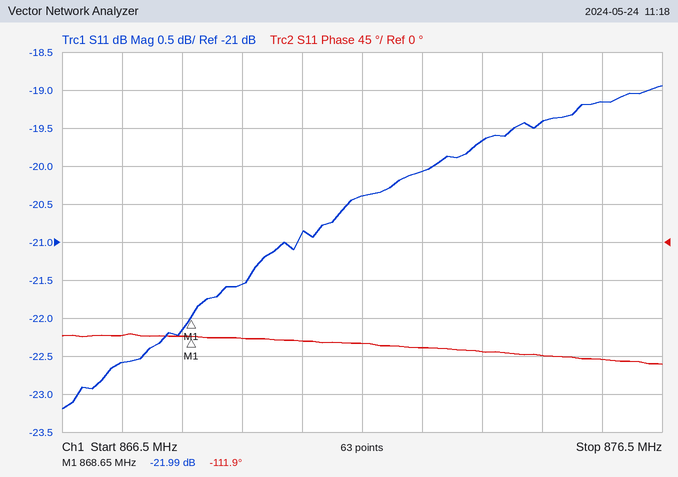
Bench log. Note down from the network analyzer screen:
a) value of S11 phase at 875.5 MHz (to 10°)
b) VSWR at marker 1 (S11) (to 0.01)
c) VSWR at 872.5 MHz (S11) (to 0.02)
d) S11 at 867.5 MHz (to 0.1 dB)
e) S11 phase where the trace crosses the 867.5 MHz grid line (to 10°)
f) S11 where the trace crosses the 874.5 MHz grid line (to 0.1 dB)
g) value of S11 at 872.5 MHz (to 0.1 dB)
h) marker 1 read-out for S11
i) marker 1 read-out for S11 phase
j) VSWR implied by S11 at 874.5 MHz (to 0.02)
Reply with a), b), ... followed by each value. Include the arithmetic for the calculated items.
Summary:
a) -140°
b) (1 + 0.0795)/(1 − 0.0795) ≈ 1.17
c) |Γ| = 10^(-20.1/20) = 0.0989; VSWR = (1 + 0.0989)/(1 − 0.0989) ≈ 1.22
d) -22.6 dB
e) -110°
f) -19.4 dB
g) -20.1 dB
h) -21.99 dB
i) -111.9°
j) |Γ| = 10^(-19.4/20) = 0.1072; VSWR = (1 + 0.1072)/(1 − 0.1072) ≈ 1.24
